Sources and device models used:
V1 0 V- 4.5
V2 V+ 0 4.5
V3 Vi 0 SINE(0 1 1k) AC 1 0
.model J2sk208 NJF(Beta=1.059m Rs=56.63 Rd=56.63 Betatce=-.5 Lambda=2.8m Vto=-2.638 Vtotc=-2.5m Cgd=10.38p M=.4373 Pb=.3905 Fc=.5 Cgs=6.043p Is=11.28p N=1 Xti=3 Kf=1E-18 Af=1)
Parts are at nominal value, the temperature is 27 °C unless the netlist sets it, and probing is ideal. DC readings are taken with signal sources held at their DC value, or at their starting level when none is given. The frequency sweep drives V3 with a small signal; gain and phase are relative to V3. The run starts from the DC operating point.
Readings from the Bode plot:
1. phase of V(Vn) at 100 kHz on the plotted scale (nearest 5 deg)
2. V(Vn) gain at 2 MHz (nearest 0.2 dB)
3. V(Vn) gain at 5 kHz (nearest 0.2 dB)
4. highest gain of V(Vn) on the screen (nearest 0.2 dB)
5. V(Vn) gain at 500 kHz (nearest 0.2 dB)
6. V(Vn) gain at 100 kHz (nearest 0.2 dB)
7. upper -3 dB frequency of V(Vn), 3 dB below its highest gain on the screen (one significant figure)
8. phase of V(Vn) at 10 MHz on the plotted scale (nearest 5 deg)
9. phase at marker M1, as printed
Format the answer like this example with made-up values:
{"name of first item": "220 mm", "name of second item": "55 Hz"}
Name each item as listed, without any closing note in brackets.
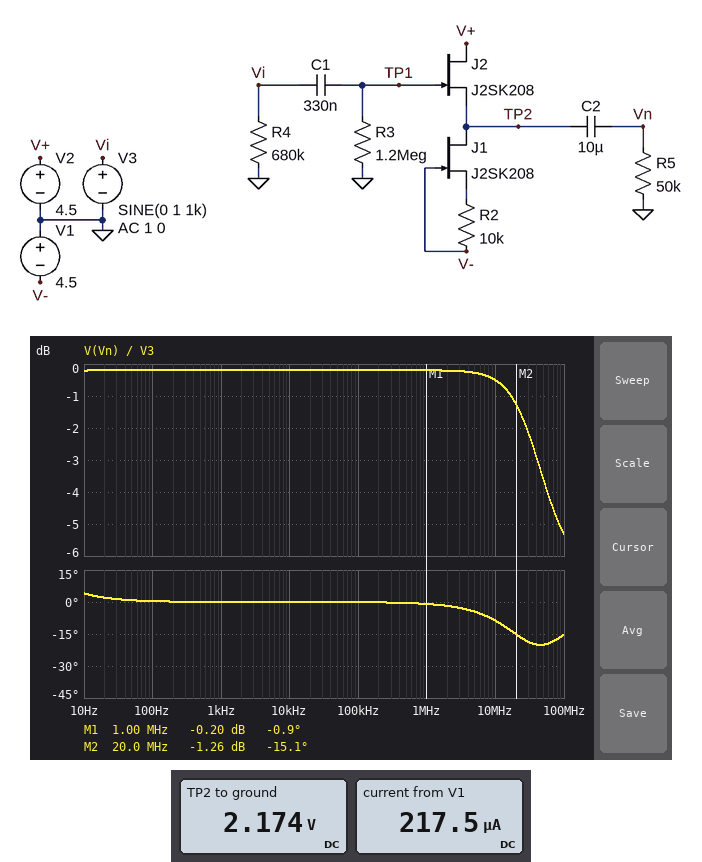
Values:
{"phase of V(Vn) at 100 kHz on the plotted scale": "0 deg", "V(Vn) gain at 2 MHz": "-0.2 dB", "V(Vn) gain at 5 kHz": "-0.2 dB", "highest gain of V(Vn) on the screen": "-0.2 dB", "V(Vn) gain at 500 kHz": "-0.2 dB", "V(Vn) gain at 100 kHz": "-0.2 dB", "upper -3 dB frequency of V(Vn), 3 dB below its highest gain on the screen": "40 MHz", "phase of V(Vn) at 10 MHz on the plotted scale": "-10 deg", "phase at marker M1, as printed": "-0.9 deg"}
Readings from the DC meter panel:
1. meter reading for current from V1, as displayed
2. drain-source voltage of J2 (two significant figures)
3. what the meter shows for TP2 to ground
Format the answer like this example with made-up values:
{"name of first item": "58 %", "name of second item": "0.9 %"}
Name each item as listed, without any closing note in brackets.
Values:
{"meter reading for current from V1, as displayed": "217.5 µA", "drain-source voltage of J2": "2.3 V", "what the meter shows for TP2 to ground": "2.174 V"}
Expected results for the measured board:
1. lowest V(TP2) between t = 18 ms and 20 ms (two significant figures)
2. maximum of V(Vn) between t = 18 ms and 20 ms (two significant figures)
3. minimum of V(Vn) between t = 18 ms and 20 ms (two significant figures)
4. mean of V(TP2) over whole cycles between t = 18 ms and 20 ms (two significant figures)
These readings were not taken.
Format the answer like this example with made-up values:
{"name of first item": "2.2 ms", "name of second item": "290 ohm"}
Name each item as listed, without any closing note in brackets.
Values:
{"lowest V(TP2) between t = 18 ms and 20 ms": "1.2 V", "maximum of V(Vn) between t = 18 ms and 20 ms": "980 mV", "minimum of V(Vn) between t = 18 ms and 20 ms": "-980 mV", "mean of V(TP2) over whole cycles between t = 18 ms and 20 ms": "2.2 V"}
